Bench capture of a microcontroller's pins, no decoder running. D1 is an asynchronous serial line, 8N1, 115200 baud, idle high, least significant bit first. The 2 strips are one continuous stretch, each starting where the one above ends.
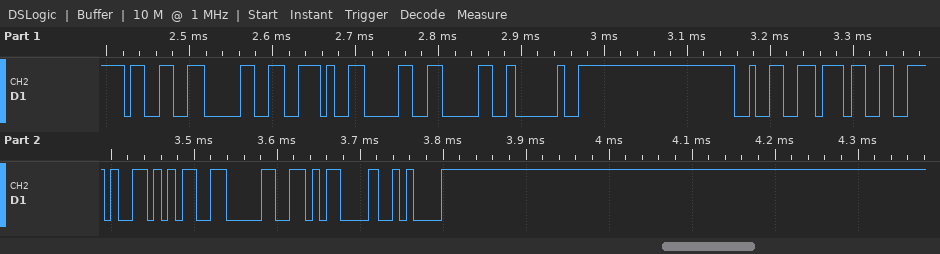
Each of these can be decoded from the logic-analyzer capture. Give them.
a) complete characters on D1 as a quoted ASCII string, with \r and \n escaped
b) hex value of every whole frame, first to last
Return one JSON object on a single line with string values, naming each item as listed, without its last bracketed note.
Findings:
{"complete characters on D1 as a quoted ASCII string, with \\r and \\n escaped": "\"30.00 27.50\\r\\n\"", "hex value of every whole frame, first to last": "0x33 0x30 0x2E 0x30 0x30 0x20 0x32 0x37 0x2E 0x35 0x30 0x0D 0x0A"}
